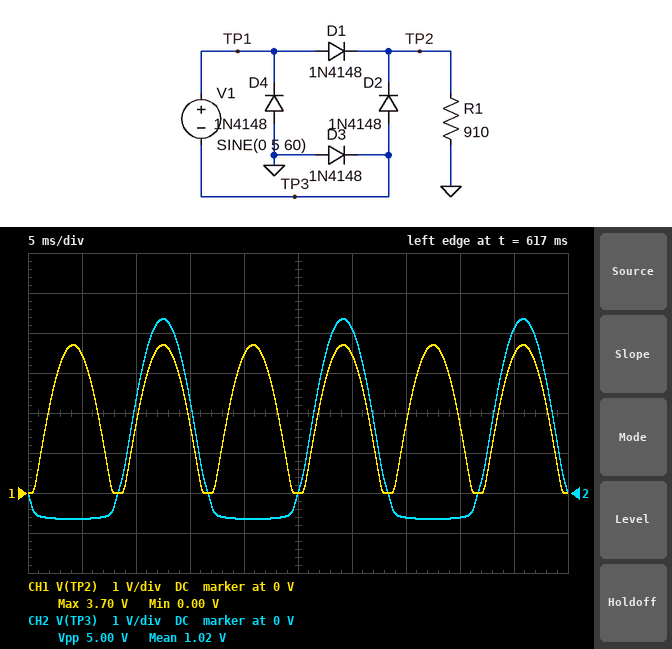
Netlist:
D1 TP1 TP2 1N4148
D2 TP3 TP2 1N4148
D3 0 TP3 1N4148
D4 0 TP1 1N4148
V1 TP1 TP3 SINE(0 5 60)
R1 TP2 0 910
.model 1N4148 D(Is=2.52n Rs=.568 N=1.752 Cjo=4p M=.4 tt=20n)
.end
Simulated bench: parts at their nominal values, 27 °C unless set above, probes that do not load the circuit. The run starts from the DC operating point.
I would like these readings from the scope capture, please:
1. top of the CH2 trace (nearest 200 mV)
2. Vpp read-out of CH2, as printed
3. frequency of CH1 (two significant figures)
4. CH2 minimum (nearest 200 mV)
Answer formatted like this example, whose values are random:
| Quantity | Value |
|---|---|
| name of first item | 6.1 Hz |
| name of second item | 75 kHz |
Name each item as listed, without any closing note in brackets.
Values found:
| Quantity | Value |
|---|---|
| top of the CH2 trace | 4.4 V |
| Vpp read-out of CH2, as printed | 5.00 V |
| frequency of CH1 | 120 Hz |
| CH2 minimum | -600 mV |
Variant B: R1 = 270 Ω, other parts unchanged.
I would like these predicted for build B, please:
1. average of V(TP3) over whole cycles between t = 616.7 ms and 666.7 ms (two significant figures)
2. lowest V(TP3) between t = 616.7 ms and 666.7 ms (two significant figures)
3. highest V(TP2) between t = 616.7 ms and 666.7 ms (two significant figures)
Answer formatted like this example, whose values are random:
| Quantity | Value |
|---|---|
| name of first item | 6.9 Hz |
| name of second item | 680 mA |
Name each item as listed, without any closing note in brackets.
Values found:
| Quantity | Value |
|---|---|
| average of V(TP3) over whole cycles between t = 616.7 ms and 666.7 ms | 970 mV |
| lowest V(TP3) between t = 616.7 ms and 666.7 ms | -710 mV |
| highest V(TP2) between t = 616.7 ms and 666.7 ms | 3.6 V |
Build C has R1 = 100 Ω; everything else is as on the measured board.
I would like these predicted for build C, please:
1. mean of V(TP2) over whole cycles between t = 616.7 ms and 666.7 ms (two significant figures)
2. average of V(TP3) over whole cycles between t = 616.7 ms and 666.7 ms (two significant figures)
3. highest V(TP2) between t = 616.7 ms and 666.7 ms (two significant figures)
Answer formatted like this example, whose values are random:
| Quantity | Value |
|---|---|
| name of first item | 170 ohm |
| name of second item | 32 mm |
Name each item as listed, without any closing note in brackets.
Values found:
| Quantity | Value |
|---|---|
| mean of V(TP2) over whole cycles between t = 616.7 ms and 666.7 ms | 1.9 V |
| average of V(TP3) over whole cycles between t = 616.7 ms and 666.7 ms | 930 mV |
| highest V(TP2) between t = 616.7 ms and 666.7 ms | 3.5 V |
